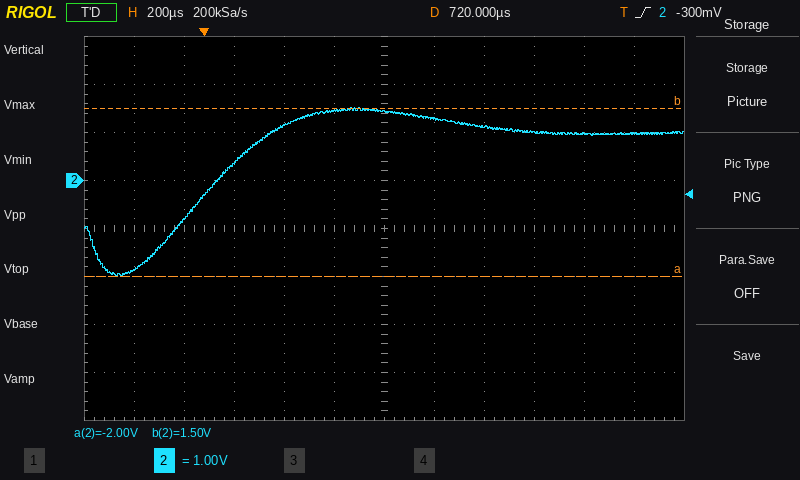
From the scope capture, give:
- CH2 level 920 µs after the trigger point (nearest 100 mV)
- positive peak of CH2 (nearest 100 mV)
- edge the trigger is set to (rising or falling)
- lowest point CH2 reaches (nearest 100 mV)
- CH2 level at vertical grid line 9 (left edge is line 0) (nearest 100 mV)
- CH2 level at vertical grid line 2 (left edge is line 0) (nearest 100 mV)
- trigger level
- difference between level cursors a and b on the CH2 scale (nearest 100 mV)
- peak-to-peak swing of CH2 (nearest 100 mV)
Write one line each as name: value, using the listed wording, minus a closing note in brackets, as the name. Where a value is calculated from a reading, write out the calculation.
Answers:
CH2 level 920 µs after the trigger point: 1.3 V
positive peak of CH2: 1.5 V
edge the trigger is set to: rising
lowest point CH2 reaches: -2.0 V
CH2 level at vertical grid line 9 (left edge is line 0): 1.0 V
CH2 level at vertical grid line 2 (left edge is line 0): -800 mV
trigger level: -300 mV
difference between level cursors a and b on the CH2 scale: 3.5 V
peak-to-peak swing of CH2: 1.5 V − (-2.0 V) = 3.5 V
